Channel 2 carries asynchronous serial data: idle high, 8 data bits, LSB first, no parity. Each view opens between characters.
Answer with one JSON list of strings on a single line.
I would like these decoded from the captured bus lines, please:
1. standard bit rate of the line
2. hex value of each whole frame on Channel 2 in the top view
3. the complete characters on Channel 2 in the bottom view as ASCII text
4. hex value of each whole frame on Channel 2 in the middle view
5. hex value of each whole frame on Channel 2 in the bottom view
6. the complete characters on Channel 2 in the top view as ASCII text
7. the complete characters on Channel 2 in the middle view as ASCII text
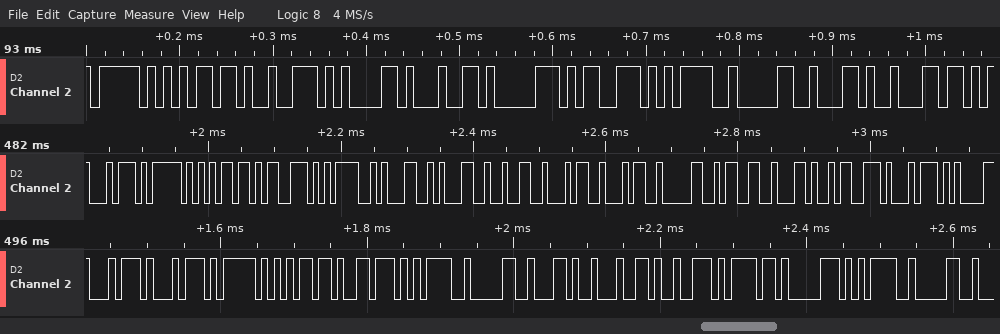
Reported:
["115200 baud", "5F, 6D, 72, 61, 64, 70, 73, 3D, 30, 2C, 6C", "\"tt_mv=0,drop=0\"", "74, 5F, 6D, 73, 3D, 31, 31, 32, 34, 34, 30, 33, 2C, 73, 74", "74, 74, 5F, 6D, 76, 3D, 30, 2C, 64, 72, 6F, 70, 3D, 30", "\"_mradps=0,l\"", "\"t_ms=1124403,st\""]
